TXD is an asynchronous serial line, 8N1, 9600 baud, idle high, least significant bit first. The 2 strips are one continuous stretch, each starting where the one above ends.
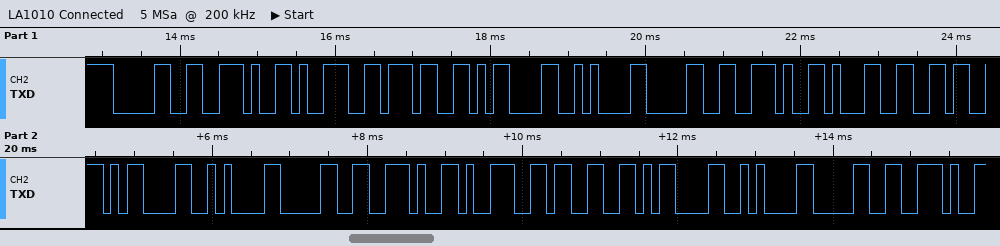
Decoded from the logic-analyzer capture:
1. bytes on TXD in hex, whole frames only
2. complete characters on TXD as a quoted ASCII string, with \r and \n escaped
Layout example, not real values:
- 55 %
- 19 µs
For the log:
- 30 2E 39 37 0D 0A 30 2E 31 36 0D 0A 30 2E 39 33 0D 0A 30 2E
- "0.97\r\n0.16\r\n0.93\r\n0."
